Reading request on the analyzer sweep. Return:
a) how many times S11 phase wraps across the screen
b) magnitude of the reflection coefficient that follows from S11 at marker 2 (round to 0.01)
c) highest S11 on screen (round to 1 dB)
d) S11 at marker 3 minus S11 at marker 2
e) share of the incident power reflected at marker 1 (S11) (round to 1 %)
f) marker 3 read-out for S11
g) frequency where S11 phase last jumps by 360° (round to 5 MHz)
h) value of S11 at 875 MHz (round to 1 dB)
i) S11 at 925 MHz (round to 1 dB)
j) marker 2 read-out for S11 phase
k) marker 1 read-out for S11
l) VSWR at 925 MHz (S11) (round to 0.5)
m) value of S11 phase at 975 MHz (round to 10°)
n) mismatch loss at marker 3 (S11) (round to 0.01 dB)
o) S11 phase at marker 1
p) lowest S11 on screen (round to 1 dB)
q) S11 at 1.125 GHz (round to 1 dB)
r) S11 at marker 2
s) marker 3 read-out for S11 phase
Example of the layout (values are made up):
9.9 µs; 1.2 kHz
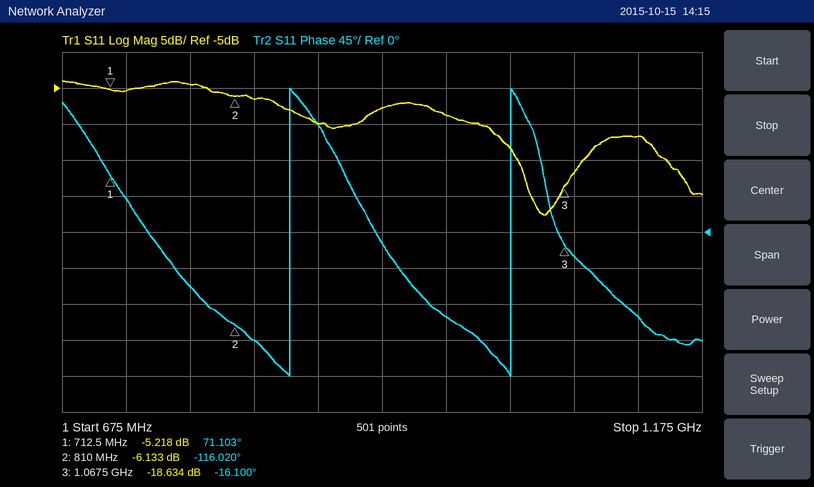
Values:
2; 0.49; -4 dB; -12.501 dB; 30 %; -18.634 dB; 1.025 GHz; -10 dB; -8 dB; -116.020°; -5.218 dB; 2.5; -110°; 0.06 dB; 71.103°; -23 dB; -12 dB; -6.133 dB; -16.100°
